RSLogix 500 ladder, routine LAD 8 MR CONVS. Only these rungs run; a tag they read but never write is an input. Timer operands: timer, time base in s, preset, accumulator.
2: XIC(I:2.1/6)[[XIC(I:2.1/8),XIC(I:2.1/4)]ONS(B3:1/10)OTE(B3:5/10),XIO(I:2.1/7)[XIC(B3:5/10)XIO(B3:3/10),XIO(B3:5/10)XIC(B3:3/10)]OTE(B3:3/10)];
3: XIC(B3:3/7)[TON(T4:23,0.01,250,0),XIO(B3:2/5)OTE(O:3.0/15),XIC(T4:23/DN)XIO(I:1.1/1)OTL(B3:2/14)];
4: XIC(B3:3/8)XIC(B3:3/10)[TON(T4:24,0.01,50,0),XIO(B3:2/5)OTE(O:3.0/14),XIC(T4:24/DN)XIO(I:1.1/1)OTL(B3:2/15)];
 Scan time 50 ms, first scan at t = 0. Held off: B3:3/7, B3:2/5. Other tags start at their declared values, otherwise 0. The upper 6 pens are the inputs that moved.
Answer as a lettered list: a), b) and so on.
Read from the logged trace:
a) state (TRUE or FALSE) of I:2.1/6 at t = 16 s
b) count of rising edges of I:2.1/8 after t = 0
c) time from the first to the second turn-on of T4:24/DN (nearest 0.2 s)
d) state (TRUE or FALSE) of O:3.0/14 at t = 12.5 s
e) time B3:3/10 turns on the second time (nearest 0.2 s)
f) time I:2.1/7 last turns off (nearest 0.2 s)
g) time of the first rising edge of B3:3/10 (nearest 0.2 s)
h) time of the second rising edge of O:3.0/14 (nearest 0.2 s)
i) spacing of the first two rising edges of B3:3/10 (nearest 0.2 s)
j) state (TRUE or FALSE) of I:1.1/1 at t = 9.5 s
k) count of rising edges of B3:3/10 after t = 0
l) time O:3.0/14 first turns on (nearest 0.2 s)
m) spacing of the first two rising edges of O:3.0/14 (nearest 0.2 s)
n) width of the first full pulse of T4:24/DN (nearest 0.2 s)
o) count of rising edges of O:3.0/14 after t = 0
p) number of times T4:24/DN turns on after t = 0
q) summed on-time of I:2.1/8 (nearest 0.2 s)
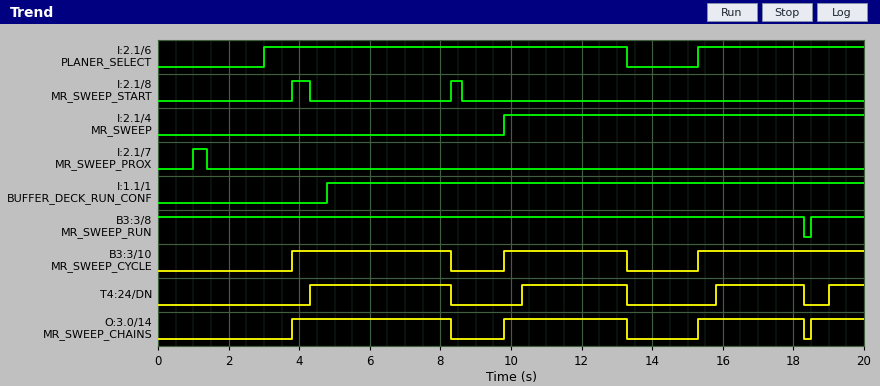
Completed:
a) TRUE
b) 2
c) 6.0 s
d) TRUE
e) 9.8 s
f) 1.4 s
g) 3.8 s
h) 9.8 s
i) 6.0 s
j) TRUE
k) 3
l) 3.8 s
m) 6.0 s
n) 4.0 s
o) 4
p) 4
q) 0.8 s
